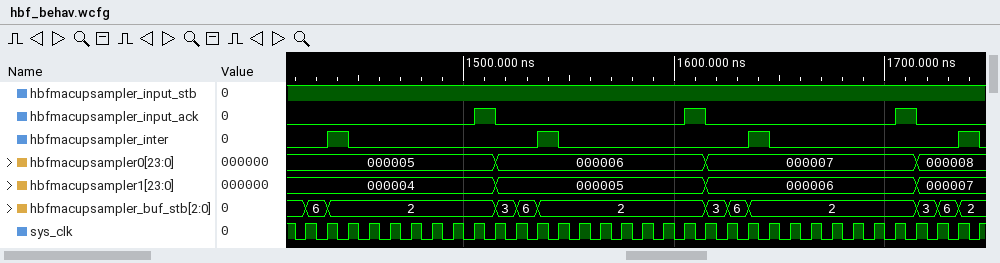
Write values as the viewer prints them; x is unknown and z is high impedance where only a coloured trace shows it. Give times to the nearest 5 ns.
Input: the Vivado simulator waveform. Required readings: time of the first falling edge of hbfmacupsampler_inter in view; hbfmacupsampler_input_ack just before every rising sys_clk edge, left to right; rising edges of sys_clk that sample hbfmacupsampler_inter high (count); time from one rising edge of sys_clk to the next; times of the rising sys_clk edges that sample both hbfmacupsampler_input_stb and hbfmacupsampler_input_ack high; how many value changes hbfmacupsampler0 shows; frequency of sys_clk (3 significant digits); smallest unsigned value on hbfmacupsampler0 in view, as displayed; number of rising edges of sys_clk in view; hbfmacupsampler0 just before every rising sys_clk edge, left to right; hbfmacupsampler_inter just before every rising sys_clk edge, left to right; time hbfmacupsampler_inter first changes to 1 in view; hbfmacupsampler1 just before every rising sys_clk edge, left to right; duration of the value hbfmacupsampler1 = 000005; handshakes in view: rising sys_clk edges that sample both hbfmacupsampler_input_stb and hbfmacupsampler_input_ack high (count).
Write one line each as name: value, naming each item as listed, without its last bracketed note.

time of the first falling edge of hbfmacupsampler_inter in view: 1445 ns
hbfmacupsampler_input_ack just before every rising sys_clk edge, left to right: 0 0 0 0 0 0 0 0 0 1 0 0 0 0 0 0 0 0 0 1 0 0 0 0 0 0 0 0 0 1 0 0 0
rising edges of sys_clk that sample hbfmacupsampler_inter high: 4
time from one rising edge of sys_clk to the next: 10 ns
times of the rising sys_clk edges that sample both hbfmacupsampler_input_stb and hbfmacupsampler_input_ack high: 1515 ns, 1615 ns, 1715 ns
how many value changes hbfmacupsampler0 shows: 3
frequency of sys_clk: 100 MHz
smallest unsigned value on hbfmacupsampler0 in view, as displayed: 000005
number of rising edges of sys_clk in view: 33
hbfmacupsampler0 just before every rising sys_clk edge, left to right: 000005, 000005, 000005, 000005, 000005, 000005, 000005, 000005, 000005, 000005, 000006, 000006, 000006, 000006, 000006, 000006, 000006, 000006, 000006, 000006, 000007, 000007, 000007, 000007, 000007, 000007, 000007, 000007, 000007, 000007, 000008, 000008, 000008
hbfmacupsampler_inter just before every rising sys_clk edge, left to right: 0 0 1 0 0 0 0 0 0 0 0 0 1 0 0 0 0 0 0 0 0 0 1 0 0 0 0 0 0 0 0 0 1
time hbfmacupsampler_inter first changes to 1 in view: 1435 ns
hbfmacupsampler1 just before every rising sys_clk edge, left to right: 000004, 000004, 000004, 000004, 000004, 000004, 000004, 000004, 000004, 000004, 000005, 000005, 000005, 000005, 000005, 000005, 000005, 000005, 000005, 000005, 000006, 000006, 000006, 000006, 000006, 000006, 000006, 000006, 000006, 000006, 000007, 000007, 000007
duration of the value hbfmacupsampler1 = 000005: 100 ns
handshakes in view: rising sys_clk edges that sample both hbfmacupsampler_input_stb and hbfmacupsampler_input_ack high: 3
